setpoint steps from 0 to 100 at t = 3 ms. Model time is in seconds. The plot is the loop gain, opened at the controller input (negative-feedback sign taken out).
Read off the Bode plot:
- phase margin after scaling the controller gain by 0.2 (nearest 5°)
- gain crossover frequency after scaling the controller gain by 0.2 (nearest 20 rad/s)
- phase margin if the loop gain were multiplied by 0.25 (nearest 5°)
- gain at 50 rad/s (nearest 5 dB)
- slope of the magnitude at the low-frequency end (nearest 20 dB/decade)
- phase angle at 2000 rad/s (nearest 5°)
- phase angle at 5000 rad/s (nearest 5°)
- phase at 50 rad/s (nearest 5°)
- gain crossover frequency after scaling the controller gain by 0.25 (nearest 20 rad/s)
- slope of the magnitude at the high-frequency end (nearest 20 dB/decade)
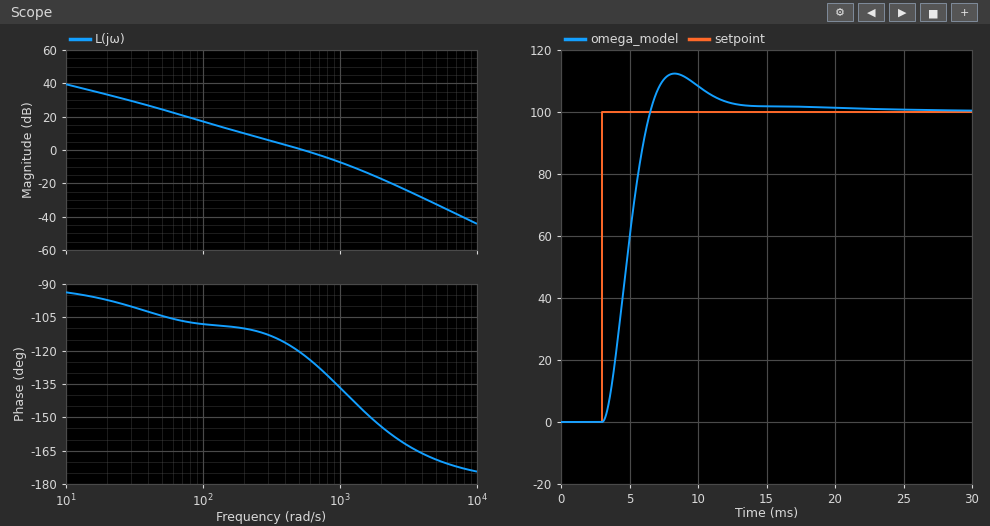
70°
140 rad/s
70°
25 dB
-20 dB/decade
-155°
-170°
-105°
160 rad/s
-40 dB/decade
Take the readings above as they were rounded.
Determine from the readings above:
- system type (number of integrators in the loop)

1
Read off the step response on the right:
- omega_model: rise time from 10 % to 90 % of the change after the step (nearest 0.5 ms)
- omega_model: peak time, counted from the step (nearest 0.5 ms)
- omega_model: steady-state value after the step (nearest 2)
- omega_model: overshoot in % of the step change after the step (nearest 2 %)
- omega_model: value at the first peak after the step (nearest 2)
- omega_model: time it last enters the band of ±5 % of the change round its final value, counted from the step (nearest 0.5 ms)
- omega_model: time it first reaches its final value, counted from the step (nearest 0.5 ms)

2.5 ms
5.5 ms
100
12 %
112
8.0 ms
3.5 ms
